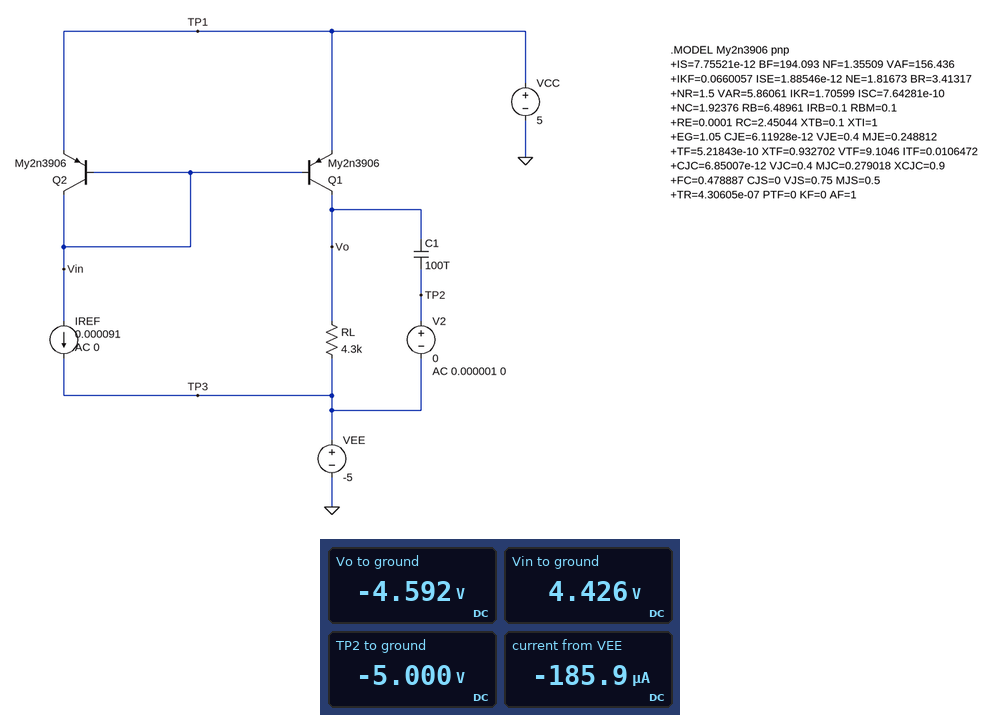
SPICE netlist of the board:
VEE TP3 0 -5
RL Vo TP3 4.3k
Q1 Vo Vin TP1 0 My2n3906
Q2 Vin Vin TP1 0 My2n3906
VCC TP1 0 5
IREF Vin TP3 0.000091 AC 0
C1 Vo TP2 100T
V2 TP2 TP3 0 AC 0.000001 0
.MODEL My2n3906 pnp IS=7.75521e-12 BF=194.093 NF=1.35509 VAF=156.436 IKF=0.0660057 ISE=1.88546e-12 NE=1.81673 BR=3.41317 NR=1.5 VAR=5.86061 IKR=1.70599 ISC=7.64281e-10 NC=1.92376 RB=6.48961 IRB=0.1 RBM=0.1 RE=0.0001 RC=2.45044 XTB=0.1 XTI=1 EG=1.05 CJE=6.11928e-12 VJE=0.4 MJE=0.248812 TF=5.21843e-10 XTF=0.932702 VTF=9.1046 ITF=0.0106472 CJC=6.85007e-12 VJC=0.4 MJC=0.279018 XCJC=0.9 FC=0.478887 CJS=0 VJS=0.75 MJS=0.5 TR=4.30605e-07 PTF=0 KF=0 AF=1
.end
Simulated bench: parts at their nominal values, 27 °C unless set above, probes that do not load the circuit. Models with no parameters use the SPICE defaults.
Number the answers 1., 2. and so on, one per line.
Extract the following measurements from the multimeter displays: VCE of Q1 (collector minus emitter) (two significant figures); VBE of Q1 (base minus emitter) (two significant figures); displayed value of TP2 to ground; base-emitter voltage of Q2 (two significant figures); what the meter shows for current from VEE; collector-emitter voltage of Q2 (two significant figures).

1. -9.6 V
2. -570 mV
3. -5.000 V
4. -570 mV
5. -185.9 µA
6. -570 mV
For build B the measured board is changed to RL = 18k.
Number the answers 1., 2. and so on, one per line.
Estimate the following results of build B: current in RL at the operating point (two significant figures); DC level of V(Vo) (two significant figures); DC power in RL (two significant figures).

1. 94 µA
2. -3.3 V
3. 160 µW
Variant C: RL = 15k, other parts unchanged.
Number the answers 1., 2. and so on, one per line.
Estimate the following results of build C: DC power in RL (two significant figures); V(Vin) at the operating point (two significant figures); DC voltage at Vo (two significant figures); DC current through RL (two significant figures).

1. 130 µW
2. 4.4 V
3. -3.6 V
4. 94 µA
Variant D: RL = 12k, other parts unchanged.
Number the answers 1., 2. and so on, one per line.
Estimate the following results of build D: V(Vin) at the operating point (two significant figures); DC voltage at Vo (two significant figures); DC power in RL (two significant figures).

1. 4.4 V
2. -3.9 V
3. 110 µW
